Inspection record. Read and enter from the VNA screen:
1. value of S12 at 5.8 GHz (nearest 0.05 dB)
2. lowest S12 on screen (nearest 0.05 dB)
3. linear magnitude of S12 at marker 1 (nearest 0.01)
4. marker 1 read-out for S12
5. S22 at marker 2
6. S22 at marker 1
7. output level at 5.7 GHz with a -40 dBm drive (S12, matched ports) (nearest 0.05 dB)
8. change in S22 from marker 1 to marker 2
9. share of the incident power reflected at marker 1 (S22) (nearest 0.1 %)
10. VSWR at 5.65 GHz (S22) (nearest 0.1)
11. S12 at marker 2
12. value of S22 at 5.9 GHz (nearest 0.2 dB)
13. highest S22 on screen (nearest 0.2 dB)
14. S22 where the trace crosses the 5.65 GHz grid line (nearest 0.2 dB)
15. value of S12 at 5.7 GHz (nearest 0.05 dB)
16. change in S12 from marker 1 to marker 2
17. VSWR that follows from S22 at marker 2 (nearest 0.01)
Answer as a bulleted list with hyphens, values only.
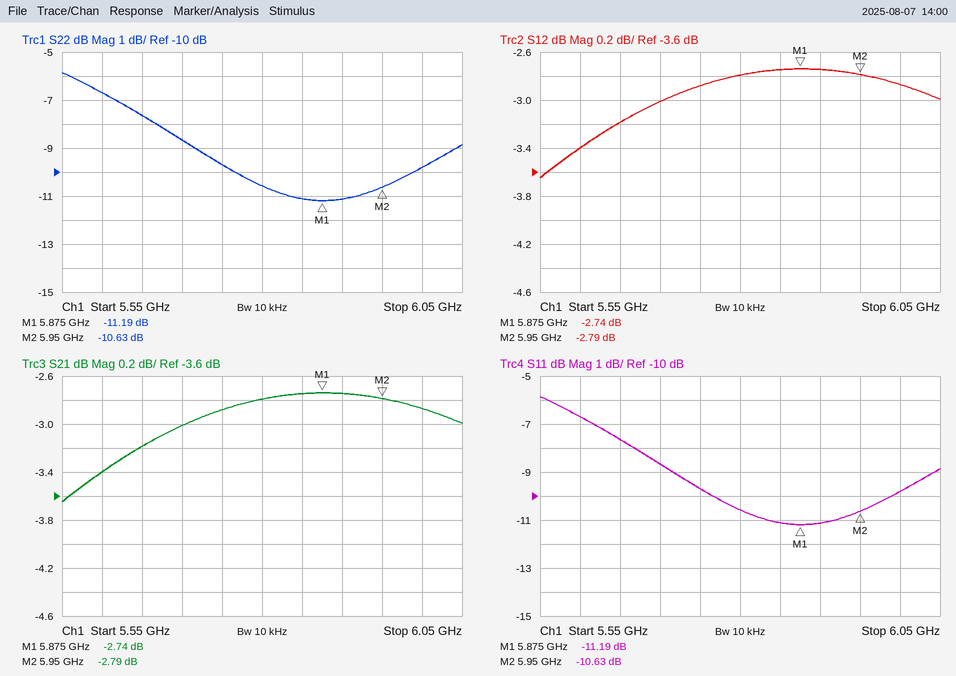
- -2.80 dB
- -3.65 dB
- 0.73
- -2.74 dB
- -10.63 dB
- -11.19 dB
- -43.00 dBm
- 0.56 dB
- 7.6 %
- 2.4
- -2.79 dB
- -11.2 dB
- -5.8 dB
- -7.6 dB
- -3.00 dB
- -0.05 dB
- 1.83
